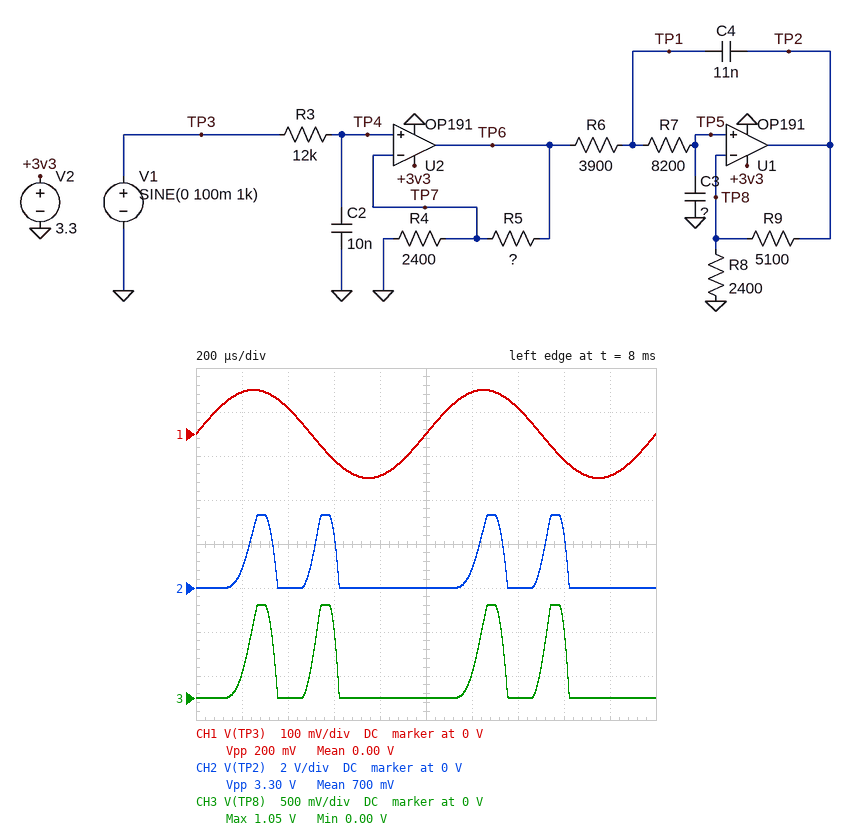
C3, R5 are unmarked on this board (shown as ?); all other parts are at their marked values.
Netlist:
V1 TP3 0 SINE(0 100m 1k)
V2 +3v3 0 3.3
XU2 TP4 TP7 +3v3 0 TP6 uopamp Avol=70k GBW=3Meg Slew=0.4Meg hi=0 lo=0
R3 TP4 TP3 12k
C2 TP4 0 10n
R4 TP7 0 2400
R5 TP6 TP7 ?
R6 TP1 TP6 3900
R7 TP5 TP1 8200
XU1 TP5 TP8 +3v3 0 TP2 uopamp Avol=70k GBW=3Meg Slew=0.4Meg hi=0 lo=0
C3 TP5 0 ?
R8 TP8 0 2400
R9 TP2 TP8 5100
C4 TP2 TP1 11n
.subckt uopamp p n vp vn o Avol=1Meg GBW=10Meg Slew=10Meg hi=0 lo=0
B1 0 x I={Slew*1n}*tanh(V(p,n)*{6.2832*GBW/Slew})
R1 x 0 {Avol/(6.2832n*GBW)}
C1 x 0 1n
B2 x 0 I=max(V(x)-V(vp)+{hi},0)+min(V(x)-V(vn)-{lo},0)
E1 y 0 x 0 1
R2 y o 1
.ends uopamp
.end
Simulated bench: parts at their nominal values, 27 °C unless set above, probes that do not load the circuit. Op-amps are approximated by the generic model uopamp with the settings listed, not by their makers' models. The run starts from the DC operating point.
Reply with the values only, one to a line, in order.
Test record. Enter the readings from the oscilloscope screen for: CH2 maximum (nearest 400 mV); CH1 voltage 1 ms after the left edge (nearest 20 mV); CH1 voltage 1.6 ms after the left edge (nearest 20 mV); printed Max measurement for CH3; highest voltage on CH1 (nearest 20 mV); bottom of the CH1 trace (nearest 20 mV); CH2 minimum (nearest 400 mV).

3.2 V
0 V
-60 mV
1.05 V
100 mV
-100 mV
0 V
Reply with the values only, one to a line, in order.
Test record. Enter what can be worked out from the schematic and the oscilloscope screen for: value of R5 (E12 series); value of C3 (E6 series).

10 kΩ
4.7 nF
